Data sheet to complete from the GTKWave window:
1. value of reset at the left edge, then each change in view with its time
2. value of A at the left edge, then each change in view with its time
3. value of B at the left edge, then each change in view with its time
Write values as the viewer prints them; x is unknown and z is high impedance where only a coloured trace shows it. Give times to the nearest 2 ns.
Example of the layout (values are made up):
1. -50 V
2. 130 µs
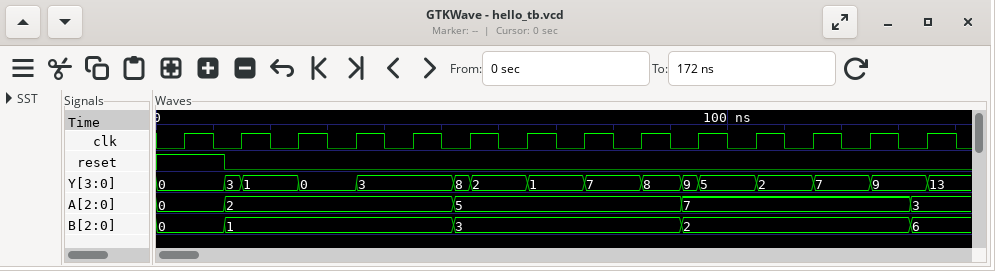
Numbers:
1. 1, 0 at 12 ns
2. 0, 2 at 12 ns, 5 at 52 ns, 7 at 92 ns, 3 at 132 ns
3. 0, 1 at 12 ns, 3 at 52 ns, 2 at 92 ns, 6 at 132 ns
